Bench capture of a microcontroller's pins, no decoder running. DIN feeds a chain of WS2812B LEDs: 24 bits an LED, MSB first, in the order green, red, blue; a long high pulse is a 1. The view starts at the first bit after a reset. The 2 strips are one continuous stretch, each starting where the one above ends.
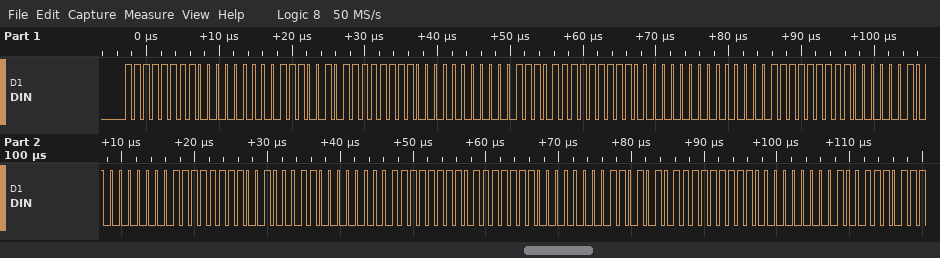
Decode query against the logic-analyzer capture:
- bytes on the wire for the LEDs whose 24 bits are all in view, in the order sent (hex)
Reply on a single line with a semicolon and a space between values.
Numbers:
FF 00 72 FF 00 1D FF 00 01 FF 02 00 FF 23 00 FF 7F 00 D5 FF 00
